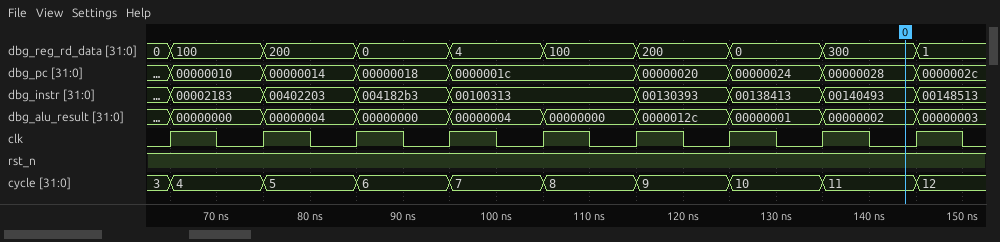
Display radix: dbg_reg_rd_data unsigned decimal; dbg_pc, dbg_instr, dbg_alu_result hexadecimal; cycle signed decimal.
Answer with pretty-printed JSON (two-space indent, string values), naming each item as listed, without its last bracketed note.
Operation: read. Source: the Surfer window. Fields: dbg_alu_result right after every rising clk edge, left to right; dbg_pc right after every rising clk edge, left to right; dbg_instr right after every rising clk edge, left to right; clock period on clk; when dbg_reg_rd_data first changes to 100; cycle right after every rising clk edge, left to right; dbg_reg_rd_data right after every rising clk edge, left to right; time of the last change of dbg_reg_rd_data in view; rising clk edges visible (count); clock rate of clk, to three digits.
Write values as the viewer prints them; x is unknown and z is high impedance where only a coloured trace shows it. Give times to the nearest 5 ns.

{
  "dbg_alu_result right after every rising clk edge, left to right": "00000000, 00000004, 00000000, 00000004, 00000000, 0000012c, 00000001, 00000002, 00000003",
  "dbg_pc right after every rising clk edge, left to right": "00000010, 00000014, 00000018, 0000001c, 0000001c, 00000020, 00000024, 00000028, 0000002c",
  "dbg_instr right after every rising clk edge, left to right": "00002183, 00402203, 004182b3, 00100313, 00100313, 00130393, 00138413, 00140493, 00148513",
  "clock period on clk": "10 ns",
  "when dbg_reg_rd_data first changes to 100": "65 ns",
  "cycle right after every rising clk edge, left to right": "4, 5, 6, 7, 8, 9, 10, 11, 12",
  "dbg_reg_rd_data right after every rising clk edge, left to right": "100, 200, 0, 4, 100, 200, 0, 300, 1",
  "time of the last change of dbg_reg_rd_data in view": "145 ns",
  "rising clk edges visible": "9",
  "clock rate of clk, to three digits": "100 MHz"
}
